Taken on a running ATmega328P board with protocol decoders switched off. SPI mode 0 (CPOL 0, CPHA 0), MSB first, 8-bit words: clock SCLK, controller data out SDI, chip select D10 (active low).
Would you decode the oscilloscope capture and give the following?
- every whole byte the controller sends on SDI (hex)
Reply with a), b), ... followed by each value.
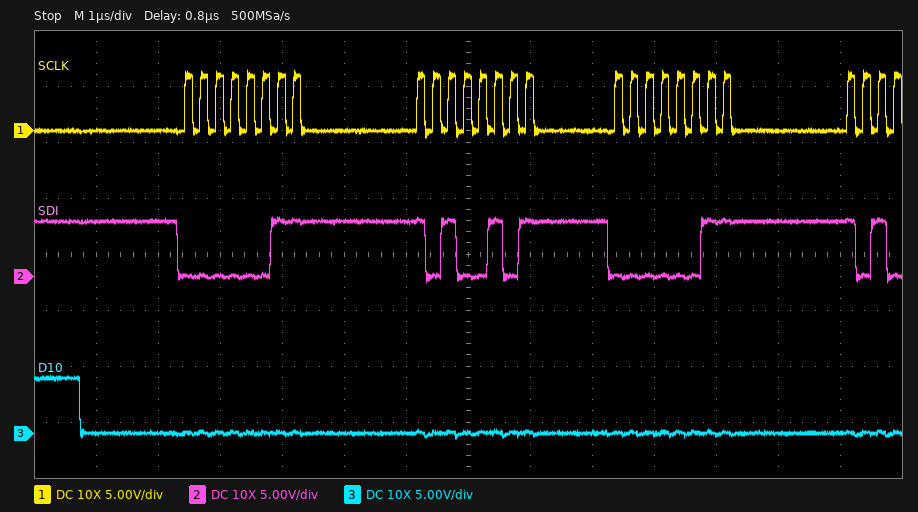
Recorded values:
a) 03 A5 03
